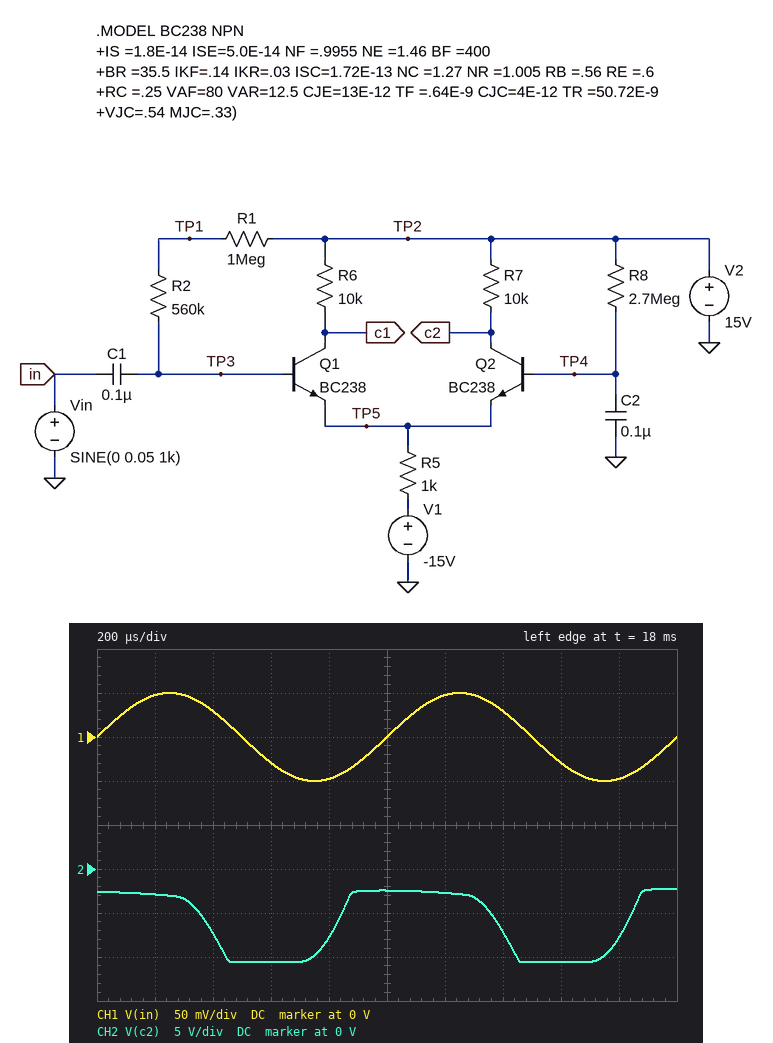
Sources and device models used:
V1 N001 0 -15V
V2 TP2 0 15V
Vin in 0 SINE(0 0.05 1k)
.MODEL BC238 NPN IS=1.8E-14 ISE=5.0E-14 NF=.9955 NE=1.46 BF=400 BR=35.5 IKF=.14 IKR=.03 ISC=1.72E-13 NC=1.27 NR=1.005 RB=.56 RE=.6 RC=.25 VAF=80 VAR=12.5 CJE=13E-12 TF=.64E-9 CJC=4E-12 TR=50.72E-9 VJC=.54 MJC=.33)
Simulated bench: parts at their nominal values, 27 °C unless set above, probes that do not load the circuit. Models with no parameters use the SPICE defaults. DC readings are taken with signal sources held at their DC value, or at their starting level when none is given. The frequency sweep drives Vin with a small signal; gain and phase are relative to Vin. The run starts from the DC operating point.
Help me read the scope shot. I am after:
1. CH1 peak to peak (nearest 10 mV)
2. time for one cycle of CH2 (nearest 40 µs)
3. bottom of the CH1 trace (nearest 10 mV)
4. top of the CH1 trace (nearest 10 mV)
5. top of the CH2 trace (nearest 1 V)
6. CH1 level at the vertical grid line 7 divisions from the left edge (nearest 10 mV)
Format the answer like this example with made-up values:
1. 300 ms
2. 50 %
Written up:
1. 100 mV
2. 1.00 ms
3. -50 mV
4. 50 mV
5. -2 V
6. 30 mV
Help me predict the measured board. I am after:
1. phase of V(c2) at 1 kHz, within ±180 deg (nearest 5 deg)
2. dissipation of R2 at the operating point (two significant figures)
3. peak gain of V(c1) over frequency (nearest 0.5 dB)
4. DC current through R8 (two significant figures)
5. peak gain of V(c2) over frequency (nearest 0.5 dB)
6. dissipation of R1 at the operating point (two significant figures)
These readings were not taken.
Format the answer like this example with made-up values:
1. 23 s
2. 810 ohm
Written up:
1. 90 deg
2. 140 µW
3. 30.0 dB
4. 9.0 µA
5. 45.5 dB
6. 240 µW
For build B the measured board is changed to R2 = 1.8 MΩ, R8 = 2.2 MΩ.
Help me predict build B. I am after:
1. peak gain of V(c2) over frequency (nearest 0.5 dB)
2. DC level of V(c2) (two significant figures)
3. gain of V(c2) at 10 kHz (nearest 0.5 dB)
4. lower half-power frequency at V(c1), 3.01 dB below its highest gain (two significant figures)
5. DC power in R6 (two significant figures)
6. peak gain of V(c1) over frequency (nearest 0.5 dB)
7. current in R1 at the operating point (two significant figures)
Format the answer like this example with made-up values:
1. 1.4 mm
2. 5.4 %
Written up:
1. 39.5 dB
2. -9.9 V
3. 36.0 dB
4. 420 kHz
5. 61 mW
6. 48.0 dB
7. 8.7 µA
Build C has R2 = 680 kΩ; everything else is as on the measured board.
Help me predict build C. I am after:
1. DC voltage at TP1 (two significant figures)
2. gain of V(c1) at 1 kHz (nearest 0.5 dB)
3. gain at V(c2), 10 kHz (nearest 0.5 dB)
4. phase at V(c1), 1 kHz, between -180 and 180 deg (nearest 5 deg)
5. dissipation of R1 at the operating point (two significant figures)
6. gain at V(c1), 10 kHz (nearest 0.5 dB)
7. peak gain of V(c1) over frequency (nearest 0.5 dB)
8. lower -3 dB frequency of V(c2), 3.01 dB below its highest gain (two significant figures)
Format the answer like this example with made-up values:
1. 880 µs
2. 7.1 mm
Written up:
1. 510 mV
2. 9.5 dB
3. 36.0 dB
4. -95 deg
5. 210 µW
6. 27.5 dB
7. 31.5 dB
8. 570 kHz
